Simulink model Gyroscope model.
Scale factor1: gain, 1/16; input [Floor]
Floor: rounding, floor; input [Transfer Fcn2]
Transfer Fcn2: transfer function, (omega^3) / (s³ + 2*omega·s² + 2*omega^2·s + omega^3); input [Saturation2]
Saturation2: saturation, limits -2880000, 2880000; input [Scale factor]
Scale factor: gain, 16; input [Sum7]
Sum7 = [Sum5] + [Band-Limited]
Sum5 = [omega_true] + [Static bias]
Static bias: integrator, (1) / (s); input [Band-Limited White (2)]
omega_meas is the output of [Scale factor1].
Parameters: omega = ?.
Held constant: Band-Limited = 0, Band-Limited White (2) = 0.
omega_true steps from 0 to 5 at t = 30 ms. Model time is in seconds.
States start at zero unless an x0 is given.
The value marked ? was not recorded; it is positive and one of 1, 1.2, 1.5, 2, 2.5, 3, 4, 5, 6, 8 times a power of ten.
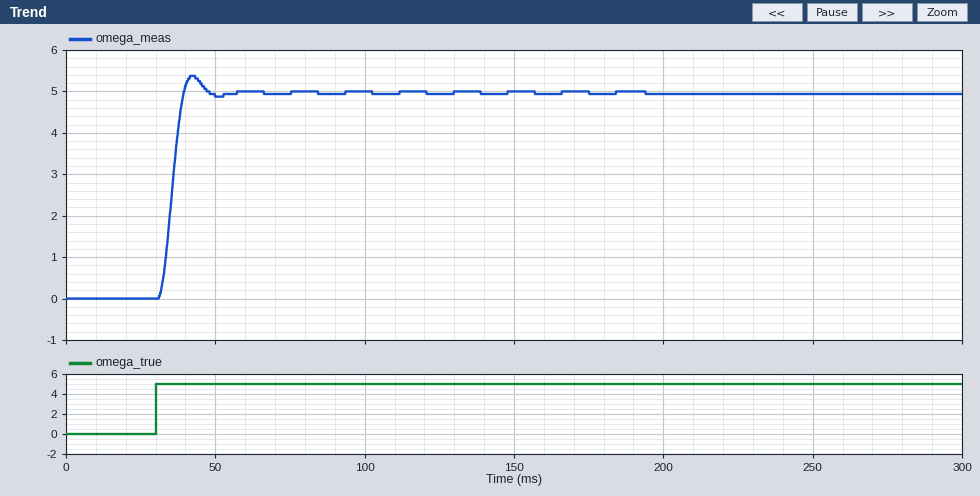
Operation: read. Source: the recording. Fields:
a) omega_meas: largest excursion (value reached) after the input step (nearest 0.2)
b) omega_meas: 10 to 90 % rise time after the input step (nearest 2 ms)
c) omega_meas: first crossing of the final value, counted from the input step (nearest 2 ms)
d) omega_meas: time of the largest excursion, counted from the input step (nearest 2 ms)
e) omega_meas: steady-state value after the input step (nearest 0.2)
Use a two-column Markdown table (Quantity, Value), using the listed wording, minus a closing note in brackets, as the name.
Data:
| Quantity | Value |
|---|---|
| omega_meas: largest excursion (value reached) after the input step | 5.4 |
| omega_meas: 10 to 90 % rise time after the input step | 6 ms |
| omega_meas: first crossing of the final value, counted from the input step | 10 ms |
| omega_meas: time of the largest excursion, counted from the input step | 12 ms |
| omega_meas: steady-state value after the input step | 5.0 |
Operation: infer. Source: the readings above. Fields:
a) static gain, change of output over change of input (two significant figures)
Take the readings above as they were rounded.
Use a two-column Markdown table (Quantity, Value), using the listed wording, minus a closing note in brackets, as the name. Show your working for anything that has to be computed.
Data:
| Quantity | Value |
|---|---|
| static gain, change of output over change of input | (5 - 0) / (5 - 0) = 1.0 |
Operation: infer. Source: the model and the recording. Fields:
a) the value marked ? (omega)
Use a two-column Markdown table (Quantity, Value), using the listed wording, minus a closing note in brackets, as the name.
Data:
| Quantity | Value |
|---|---|
| the value marked ? | 400 |
